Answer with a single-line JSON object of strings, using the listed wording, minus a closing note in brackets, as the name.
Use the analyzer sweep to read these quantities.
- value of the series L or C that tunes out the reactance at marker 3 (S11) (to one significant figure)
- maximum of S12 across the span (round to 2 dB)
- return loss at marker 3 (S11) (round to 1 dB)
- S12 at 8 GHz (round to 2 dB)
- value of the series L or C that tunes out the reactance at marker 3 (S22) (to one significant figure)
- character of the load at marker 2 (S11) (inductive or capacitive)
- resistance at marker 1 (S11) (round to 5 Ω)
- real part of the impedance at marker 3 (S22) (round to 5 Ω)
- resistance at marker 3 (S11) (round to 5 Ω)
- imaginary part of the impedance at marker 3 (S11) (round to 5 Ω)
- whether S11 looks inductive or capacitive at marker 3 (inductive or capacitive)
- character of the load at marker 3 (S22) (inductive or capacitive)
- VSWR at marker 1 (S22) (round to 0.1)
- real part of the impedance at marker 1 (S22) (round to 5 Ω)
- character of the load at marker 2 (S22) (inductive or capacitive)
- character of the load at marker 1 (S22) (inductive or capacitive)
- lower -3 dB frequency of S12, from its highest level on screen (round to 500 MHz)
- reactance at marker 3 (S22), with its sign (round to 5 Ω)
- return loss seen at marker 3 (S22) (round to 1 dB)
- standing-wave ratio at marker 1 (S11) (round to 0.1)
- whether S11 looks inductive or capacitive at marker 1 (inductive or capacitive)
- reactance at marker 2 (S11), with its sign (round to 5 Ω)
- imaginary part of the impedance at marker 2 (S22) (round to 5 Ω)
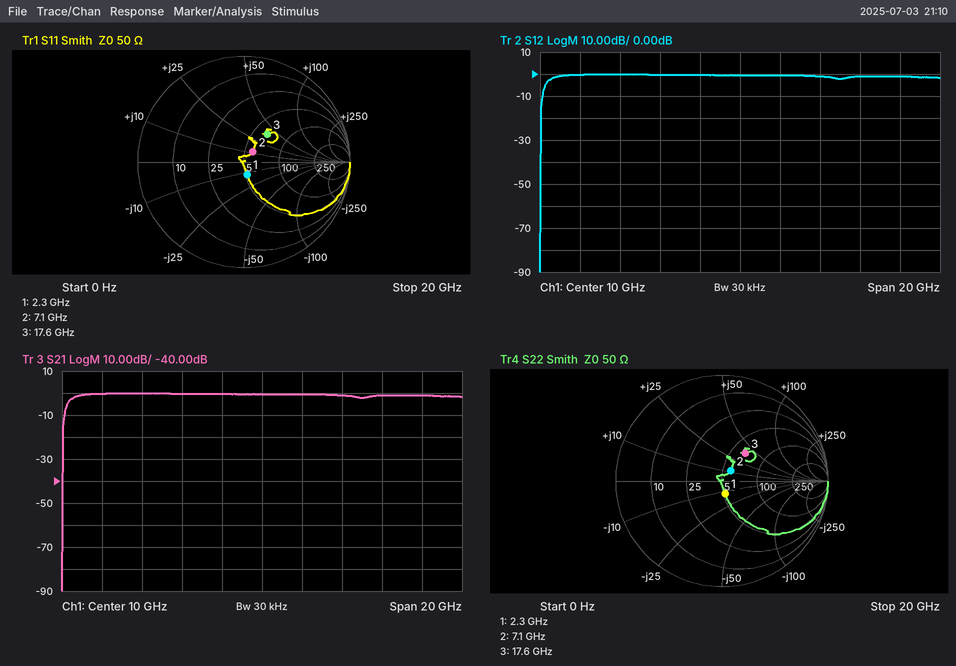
{"value of the series L or C that tunes out the reactance at marker 3 (S11)": "200 fF", "maximum of S12 across the span": "0 dB", "return loss at marker 3 (S11)": "9 dB", "S12 at 8 GHz": "0 dB", "value of the series L or C that tunes out the reactance at marker 3 (S22)": "200 fF", "character of the load at marker 2 (S11)": "inductive", "resistance at marker 1 (S11)": "50 Ω", "real part of the impedance at marker 3 (S22)": "65 Ω", "resistance at marker 3 (S11)": "65 Ω", "imaginary part of the impedance at marker 3 (S11)": "+40 Ω", "whether S11 looks inductive or capacitive at marker 3": "inductive", "character of the load at marker 3 (S22)": "inductive", "VSWR at marker 1 (S22)": "1.3", "real part of the impedance at marker 1 (S22)": "50 Ω", "character of the load at marker 2 (S22)": "inductive", "character of the load at marker 1 (S22)": "capacitive", "lower -3 dB frequency of S12, from its highest level on screen": "500 MHz", "reactance at marker 3 (S22), with its sign": "+40 Ω", "return loss seen at marker 3 (S22)": "9 dB", "standing-wave ratio at marker 1 (S11)": "1.3", "whether S11 looks inductive or capacitive at marker 1": "capacitive", "reactance at marker 2 (S11), with its sign": "+10 Ω", "imaginary part of the impedance at marker 2 (S22)": "+10 Ω"}
